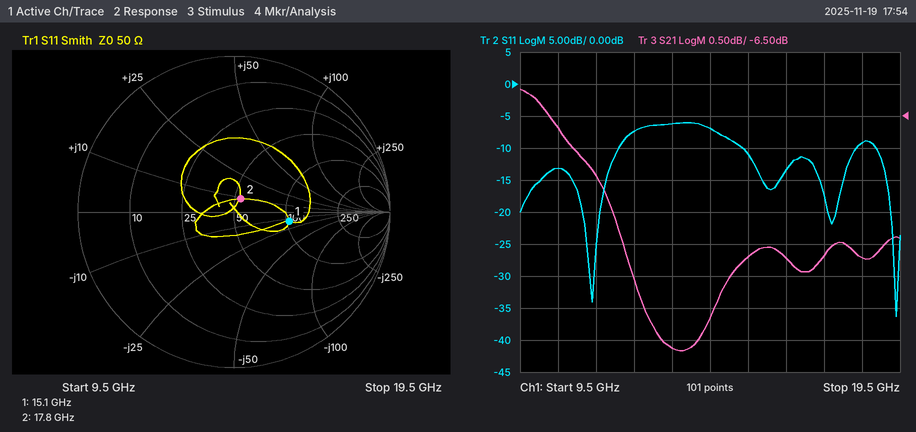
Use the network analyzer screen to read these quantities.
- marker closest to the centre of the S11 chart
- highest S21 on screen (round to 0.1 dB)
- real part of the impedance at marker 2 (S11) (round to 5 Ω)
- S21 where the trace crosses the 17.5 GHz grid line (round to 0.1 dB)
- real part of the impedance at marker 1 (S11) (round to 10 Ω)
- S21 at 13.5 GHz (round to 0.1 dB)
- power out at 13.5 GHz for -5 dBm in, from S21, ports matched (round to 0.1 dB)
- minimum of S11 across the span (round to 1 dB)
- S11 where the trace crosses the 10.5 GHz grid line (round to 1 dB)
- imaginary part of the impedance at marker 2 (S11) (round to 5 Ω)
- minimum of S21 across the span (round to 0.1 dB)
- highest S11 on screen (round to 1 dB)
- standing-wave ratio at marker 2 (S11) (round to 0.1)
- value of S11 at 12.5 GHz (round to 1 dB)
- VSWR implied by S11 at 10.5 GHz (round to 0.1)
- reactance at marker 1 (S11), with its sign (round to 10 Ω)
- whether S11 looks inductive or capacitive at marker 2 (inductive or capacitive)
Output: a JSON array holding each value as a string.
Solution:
["marker 2", "-6.1 dB", "55 Ω", "-8.7 dB", "100 Ω", "-10.1 dB", "-15.1 dBm", "-36 dB", "-13 dB", "+10 Ω", "-10.2 dB", "-6 dB", "1.2", "-7 dB", "1.6", "-10 Ω", "inductive"]
